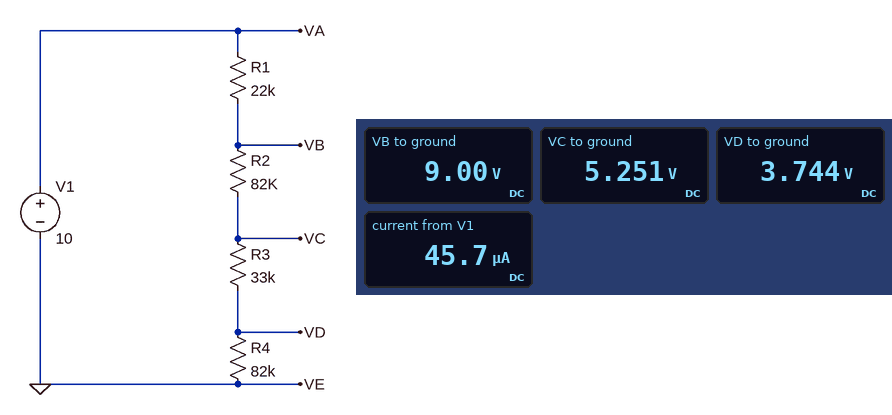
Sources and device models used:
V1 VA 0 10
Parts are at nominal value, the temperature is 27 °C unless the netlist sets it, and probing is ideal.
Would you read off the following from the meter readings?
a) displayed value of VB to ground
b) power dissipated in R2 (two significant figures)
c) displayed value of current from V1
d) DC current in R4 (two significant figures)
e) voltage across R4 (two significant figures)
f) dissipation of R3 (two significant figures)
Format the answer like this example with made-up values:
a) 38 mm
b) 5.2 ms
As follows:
a) 9.00 V
b) 170 µW
c) 45.7 µA
d) 46 µA
e) 3.7 V
f) 69 µW
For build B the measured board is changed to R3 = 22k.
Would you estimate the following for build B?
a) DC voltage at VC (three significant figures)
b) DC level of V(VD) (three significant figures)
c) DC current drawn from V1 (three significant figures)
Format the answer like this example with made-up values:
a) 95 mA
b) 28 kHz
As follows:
a) 5.00 V
b) 3.94 V
c) 48.1 µA
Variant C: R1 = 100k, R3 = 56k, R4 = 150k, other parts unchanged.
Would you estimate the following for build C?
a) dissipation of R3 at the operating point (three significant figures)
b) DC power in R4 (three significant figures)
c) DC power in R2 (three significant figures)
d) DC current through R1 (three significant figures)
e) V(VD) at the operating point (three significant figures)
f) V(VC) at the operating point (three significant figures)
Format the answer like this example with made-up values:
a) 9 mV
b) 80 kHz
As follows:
a) 37.2 µW
b) 99.6 µW
c) 54.5 µW
d) 25.8 µA
e) 3.87 V
f) 5.31 V
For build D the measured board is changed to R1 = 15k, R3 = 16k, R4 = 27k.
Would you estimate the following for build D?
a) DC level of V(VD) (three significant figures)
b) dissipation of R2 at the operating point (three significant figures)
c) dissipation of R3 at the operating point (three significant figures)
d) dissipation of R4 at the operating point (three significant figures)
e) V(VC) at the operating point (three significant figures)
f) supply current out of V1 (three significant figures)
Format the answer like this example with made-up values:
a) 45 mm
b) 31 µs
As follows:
a) 1.93 V
b) 418 µW
c) 81.6 µW
d) 138 µW
e) 3.07 V
f) 71.4 µA
